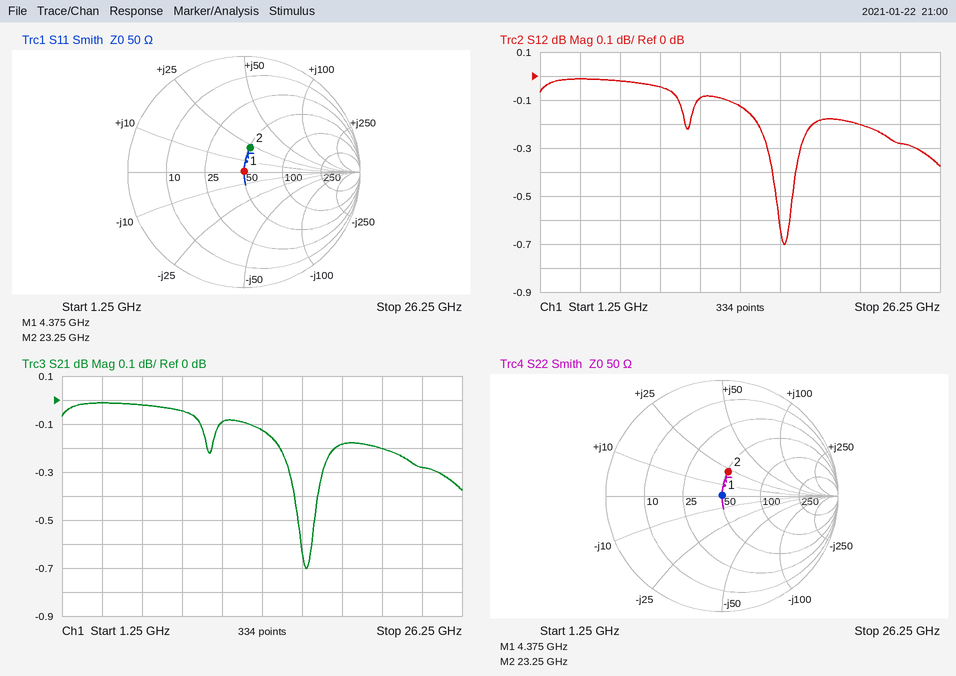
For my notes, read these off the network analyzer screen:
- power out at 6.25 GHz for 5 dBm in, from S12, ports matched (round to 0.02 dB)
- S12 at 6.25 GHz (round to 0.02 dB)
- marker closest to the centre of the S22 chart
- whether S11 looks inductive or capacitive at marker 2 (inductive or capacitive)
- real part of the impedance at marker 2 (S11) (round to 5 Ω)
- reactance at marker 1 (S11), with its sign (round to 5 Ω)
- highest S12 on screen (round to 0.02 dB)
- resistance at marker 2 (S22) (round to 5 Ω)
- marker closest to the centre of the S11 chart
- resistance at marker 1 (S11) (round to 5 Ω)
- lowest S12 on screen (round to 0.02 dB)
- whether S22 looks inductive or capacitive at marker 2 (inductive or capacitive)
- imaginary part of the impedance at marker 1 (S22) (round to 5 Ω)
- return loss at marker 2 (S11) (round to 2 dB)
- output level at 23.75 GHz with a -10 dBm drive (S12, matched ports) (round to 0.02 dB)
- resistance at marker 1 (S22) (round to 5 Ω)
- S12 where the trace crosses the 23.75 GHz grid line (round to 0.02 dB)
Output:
4.98 dBm
-0.02 dB
marker 1
inductive
50 Ω
0 Ω
-0.02 dB
50 Ω
marker 1
50 Ω
-0.70 dB
inductive
0 Ω
14 dB
-10.28 dBm
50 Ω
-0.28 dB
